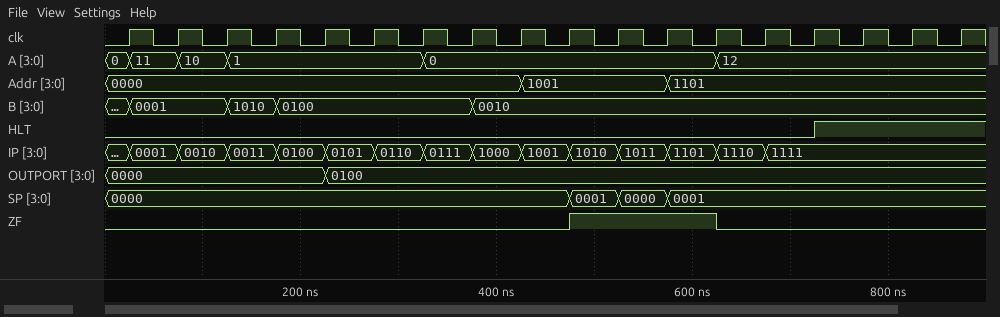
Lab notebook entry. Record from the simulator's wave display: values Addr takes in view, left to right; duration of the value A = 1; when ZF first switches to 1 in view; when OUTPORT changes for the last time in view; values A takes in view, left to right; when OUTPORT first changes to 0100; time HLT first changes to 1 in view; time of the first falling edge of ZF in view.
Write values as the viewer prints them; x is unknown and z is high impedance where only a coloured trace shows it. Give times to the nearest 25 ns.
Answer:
0000, 1001, 1101
200 ns
475 ns
225 ns
0, 11, 10, 1, 0, 12
225 ns
725 ns
625 ns
